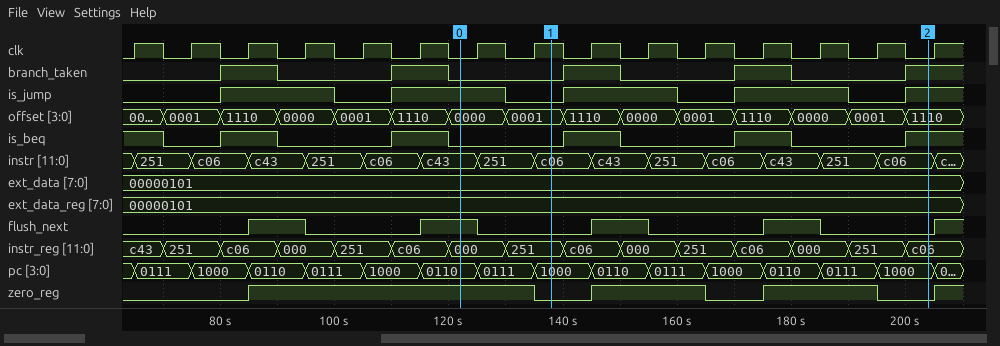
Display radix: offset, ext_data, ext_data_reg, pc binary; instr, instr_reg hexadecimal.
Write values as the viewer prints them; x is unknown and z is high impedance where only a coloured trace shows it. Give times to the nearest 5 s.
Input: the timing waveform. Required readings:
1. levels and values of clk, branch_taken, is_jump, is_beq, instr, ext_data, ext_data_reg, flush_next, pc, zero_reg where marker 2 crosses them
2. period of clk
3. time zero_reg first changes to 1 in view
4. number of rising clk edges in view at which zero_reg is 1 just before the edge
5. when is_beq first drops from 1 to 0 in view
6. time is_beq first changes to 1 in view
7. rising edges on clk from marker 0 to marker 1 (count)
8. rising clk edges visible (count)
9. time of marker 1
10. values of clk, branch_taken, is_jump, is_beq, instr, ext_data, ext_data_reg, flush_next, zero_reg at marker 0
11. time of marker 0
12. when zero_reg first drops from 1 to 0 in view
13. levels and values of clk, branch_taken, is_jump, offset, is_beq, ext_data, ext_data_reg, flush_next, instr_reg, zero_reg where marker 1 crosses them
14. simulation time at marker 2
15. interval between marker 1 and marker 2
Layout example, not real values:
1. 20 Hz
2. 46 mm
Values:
1. clk=0, branch_taken=1, is_jump=1, is_beq=1, instr=c06, ext_data=00000101, ext_data_reg=00000101, flush_next=0, pc=1000, zero_reg=0
2. 10 s
3. 85 s
4. 9
5. 70 s
6. 80 s
7. 2
8. 15
9. 140 s
10. clk=0, branch_taken=0, is_jump=1, is_beq=0, instr=c43, ext_data=00000101, ext_data_reg=00000101, flush_next=1, zero_reg=1
11. 120 s
12. 135 s
13. clk=1, branch_taken=0, is_jump=0, offset=0001, is_beq=0, ext_data=00000101, ext_data_reg=00000101, flush_next=0, instr_reg=251, zero_reg=0
14. 205 s
15. 65 s
